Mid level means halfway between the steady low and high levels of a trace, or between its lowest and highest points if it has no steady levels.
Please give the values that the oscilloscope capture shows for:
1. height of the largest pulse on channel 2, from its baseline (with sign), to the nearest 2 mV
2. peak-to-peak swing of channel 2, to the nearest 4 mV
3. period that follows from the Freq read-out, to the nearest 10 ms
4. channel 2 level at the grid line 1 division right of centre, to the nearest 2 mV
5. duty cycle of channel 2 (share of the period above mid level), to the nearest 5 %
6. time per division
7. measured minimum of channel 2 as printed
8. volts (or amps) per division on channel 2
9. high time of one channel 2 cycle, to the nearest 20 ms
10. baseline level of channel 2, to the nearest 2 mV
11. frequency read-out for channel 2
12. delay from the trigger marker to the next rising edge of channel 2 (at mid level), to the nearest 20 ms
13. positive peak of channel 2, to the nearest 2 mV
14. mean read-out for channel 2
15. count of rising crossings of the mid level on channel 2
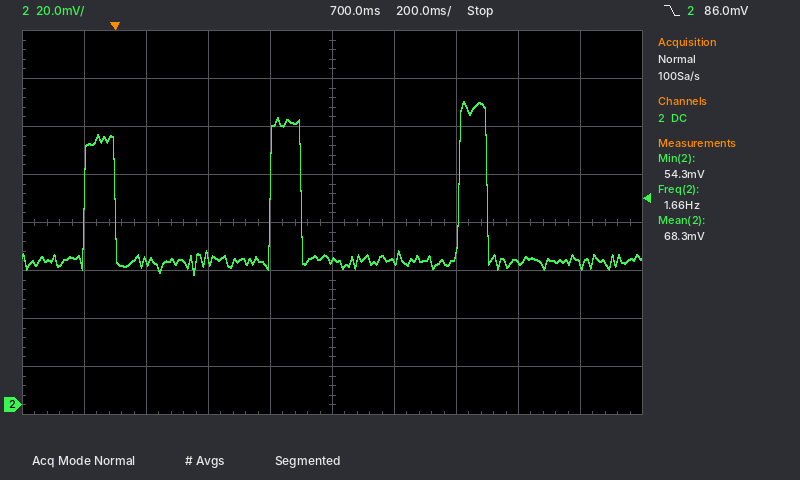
+66 mV
72 mV
600 ms
60 mV
15 %
200 ms
54.3 mV
20 mV
100 ms
60 mV
1.66 Hz
500 ms
126 mV
68.3 mV
3
